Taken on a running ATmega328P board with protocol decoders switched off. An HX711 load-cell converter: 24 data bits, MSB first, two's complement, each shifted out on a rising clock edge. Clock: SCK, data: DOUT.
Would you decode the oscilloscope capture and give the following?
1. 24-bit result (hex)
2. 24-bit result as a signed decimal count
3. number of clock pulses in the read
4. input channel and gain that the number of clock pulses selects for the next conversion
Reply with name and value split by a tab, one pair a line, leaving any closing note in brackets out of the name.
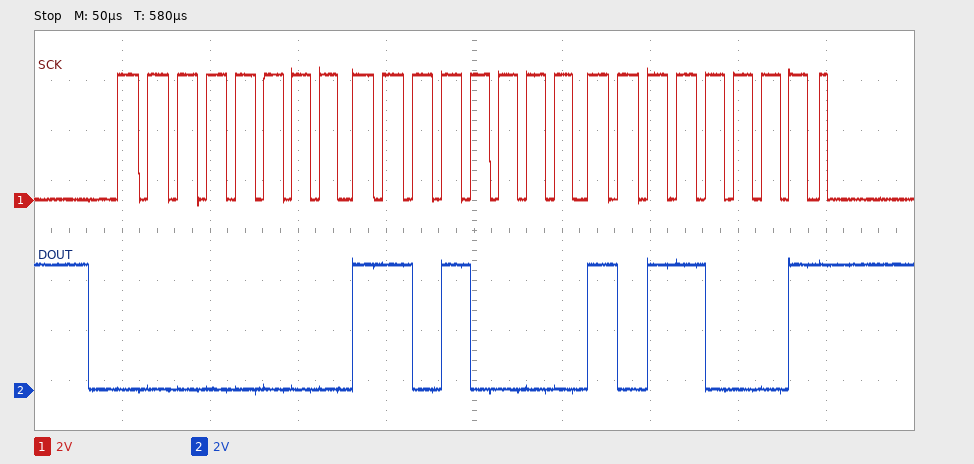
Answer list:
24-bit result	0x00D0B1
24-bit result as a signed decimal count	53425
number of clock pulses in the read	25
input channel and gain that the number of clock pulses selects for the next conversion	channel A, gain 128
